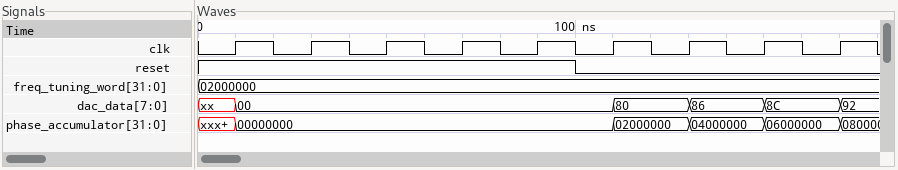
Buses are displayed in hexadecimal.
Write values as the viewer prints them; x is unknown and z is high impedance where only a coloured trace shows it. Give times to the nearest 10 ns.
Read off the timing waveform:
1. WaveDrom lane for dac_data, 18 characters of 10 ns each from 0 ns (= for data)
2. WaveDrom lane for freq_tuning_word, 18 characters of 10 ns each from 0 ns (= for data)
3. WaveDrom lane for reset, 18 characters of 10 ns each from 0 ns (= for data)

{name: 'dac_data', wave: 'x=.........=.=.=.=', data: '00 80 86 8C 92'}
{name: 'freq_tuning_word', wave: '=.................', data: '02000000'}
{name: 'reset', wave: '1.........0.......'}
